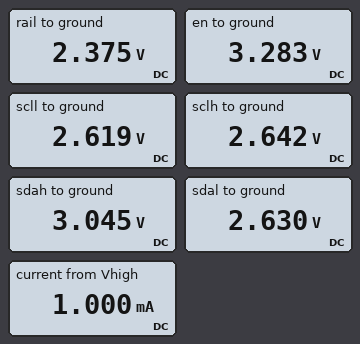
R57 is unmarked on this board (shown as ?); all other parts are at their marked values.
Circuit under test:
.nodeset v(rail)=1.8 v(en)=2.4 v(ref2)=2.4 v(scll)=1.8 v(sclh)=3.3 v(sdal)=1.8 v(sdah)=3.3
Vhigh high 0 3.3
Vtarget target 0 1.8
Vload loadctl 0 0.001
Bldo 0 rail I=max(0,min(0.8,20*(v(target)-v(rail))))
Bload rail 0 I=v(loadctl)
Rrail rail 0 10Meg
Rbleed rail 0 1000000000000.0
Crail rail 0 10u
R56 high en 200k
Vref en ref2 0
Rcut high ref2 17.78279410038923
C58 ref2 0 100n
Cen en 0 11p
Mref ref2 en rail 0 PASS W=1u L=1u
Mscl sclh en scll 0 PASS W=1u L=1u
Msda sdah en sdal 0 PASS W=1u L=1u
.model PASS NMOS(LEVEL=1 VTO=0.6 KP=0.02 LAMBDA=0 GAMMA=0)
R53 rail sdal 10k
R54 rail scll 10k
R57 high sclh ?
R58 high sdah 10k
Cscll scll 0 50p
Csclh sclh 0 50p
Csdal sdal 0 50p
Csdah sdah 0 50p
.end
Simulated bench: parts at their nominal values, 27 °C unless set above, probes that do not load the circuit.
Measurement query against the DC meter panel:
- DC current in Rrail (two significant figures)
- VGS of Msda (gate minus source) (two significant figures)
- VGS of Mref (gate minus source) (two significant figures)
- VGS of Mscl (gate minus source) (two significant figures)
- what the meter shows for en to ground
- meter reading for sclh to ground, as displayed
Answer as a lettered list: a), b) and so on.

a) 240 nA
b) 650 mV
c) 910 mV
d) 660 mV
e) 3.283 V
f) 2.642 V
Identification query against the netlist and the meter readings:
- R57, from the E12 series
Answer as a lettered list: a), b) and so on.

a) 27 kΩ
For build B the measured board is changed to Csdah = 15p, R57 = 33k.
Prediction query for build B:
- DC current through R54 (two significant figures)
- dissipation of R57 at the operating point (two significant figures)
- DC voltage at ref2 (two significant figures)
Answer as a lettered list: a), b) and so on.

a) 21 µA
b) 15 µW
c) 3.3 V
